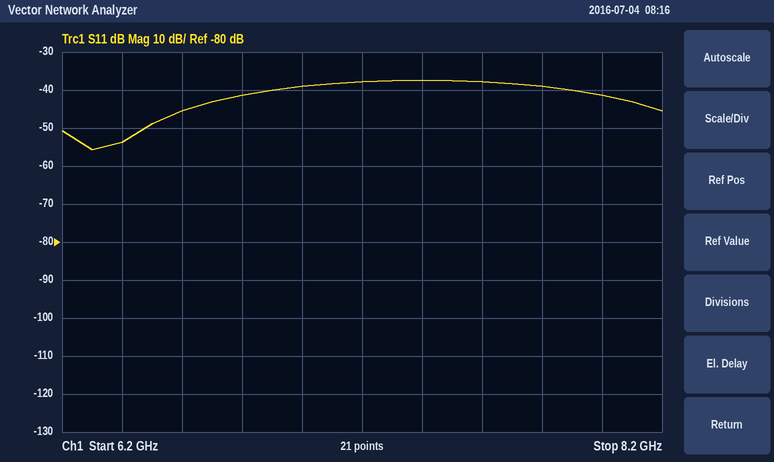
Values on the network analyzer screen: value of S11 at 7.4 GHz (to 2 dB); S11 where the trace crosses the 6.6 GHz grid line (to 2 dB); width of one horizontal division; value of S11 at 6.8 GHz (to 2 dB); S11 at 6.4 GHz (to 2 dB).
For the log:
-38 dB
-46 dB
200 MHz
-42 dB
-54 dB
